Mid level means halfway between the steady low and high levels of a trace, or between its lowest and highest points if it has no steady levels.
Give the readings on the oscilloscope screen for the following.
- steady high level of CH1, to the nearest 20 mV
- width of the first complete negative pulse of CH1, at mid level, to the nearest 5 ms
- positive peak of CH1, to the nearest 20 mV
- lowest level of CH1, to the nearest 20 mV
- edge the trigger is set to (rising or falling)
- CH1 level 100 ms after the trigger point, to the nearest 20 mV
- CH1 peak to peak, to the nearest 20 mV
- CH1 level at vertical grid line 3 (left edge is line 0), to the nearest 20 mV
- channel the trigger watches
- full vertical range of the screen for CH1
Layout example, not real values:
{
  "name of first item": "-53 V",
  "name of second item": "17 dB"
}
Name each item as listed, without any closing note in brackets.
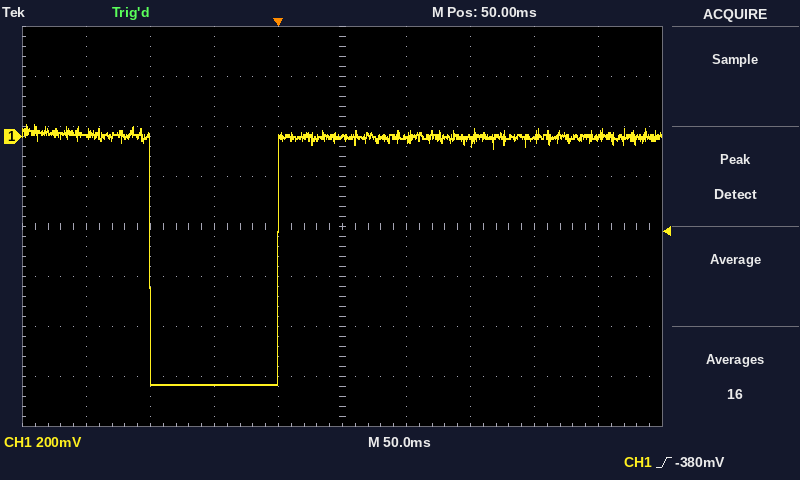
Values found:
{
  "steady high level of CH1, to the nearest 20 mV": "0 mV",
  "width of the first complete negative pulse of CH1, at mid level, to the nearest 5 ms": "100 ms",
  "positive peak of CH1, to the nearest 20 mV": "40 mV",
  "lowest level of CH1, to the nearest 20 mV": "-1.00 V",
  "edge the trigger is set to": "rising",
  "CH1 level 100 ms after the trigger point, to the nearest 20 mV": "0 mV",
  "CH1 peak to peak, to the nearest 20 mV": "1.04 V",
  "CH1 level at vertical grid line 3 (left edge is line 0), to the nearest 20 mV": "-1.00 V",
  "channel the trigger watches": "CH1",
  "full vertical range of the screen for CH1": "1.6 V"
}
